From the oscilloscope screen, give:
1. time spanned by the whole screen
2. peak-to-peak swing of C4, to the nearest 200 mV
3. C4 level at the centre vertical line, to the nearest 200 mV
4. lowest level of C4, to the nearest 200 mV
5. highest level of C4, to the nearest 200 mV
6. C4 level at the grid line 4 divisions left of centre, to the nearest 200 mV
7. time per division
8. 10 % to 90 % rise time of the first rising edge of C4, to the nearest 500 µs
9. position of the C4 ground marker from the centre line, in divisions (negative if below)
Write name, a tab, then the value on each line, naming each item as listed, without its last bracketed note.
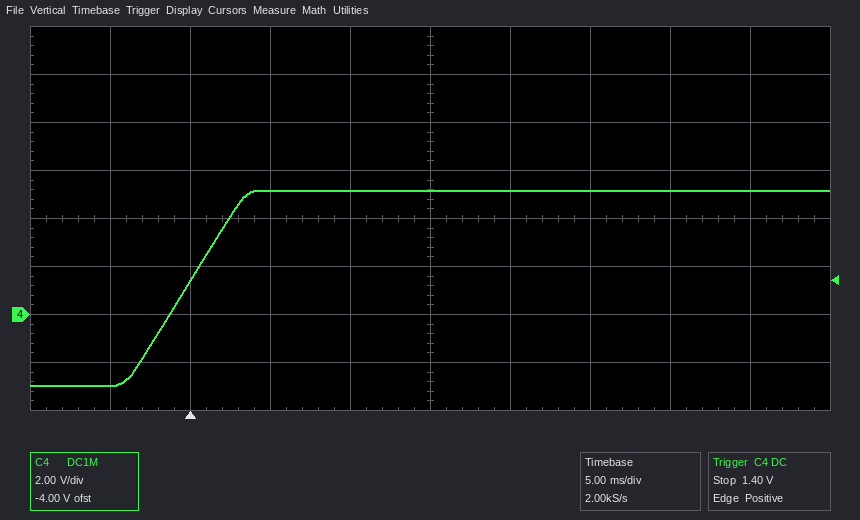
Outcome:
time spanned by the whole screen	50 ms
peak-to-peak swing of C4, to the nearest 200 mV	8.2 V
C4 level at the centre vertical line, to the nearest 200 mV	5.2 V
lowest level of C4, to the nearest 200 mV	-3.0 V
highest level of C4, to the nearest 200 mV	5.2 V
C4 level at the grid line 4 divisions left of centre, to the nearest 200 mV	-3.0 V
time per division	5 ms
10 % to 90 % rise time of the first rising edge of C4, to the nearest 500 µs	6.0 ms
position of the C4 ground marker from the centre line, in divisions	-2.0 div
